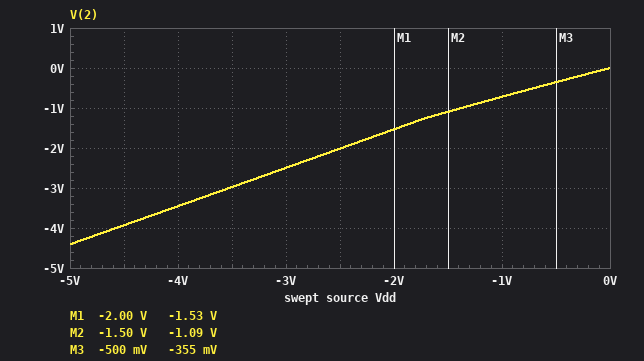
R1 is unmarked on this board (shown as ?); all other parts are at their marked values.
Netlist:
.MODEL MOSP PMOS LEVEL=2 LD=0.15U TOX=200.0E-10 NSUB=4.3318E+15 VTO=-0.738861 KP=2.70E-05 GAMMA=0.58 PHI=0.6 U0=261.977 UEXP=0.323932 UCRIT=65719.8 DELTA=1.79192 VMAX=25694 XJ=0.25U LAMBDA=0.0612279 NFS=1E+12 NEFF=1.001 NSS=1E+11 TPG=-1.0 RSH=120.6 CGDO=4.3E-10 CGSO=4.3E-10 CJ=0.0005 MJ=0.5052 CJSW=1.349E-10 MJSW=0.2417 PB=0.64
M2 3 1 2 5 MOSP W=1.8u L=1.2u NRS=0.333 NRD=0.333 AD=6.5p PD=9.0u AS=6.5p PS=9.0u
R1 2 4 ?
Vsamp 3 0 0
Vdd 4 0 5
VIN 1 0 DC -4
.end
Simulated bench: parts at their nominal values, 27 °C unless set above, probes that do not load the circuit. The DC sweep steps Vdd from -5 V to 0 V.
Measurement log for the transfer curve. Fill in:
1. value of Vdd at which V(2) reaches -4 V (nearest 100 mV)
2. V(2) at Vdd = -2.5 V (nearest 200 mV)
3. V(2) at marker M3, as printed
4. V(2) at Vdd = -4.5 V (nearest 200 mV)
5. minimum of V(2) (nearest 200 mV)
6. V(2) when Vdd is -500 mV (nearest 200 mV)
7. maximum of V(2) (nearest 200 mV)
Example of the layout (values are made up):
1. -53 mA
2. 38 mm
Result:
1. -4.6 V
2. -2.0 V
3. -355 mV
4. -4.0 V
5. -4.4 V
6. -400 mV
7. 0 V
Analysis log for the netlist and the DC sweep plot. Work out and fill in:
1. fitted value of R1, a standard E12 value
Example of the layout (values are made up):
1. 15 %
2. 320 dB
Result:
1. 4.7 kΩ
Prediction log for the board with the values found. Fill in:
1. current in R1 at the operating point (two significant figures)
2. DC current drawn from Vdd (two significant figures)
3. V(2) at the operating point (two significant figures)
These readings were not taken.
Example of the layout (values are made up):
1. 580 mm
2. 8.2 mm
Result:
1. 300 µA
2. 300 µA
3. 3.6 V
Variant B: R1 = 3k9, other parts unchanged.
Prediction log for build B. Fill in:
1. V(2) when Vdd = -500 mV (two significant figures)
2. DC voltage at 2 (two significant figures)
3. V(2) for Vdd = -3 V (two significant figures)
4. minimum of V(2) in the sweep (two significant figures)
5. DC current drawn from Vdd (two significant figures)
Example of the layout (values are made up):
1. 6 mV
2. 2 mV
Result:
1. -370 mV
2. 3.8 V
3. -2.6 V
4. -4.5 V
5. 310 µA
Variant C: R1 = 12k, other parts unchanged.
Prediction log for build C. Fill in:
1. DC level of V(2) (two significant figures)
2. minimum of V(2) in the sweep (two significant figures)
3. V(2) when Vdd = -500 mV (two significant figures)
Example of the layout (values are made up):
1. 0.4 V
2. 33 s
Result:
1. 2.4 V
2. -3.6 V
3. -240 mV
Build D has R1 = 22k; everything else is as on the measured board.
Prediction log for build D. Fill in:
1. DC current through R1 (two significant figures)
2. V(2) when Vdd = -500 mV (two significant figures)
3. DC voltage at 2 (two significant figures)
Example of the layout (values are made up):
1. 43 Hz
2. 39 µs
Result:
1. 160 µA
2. -170 mV
3. 1.5 V
